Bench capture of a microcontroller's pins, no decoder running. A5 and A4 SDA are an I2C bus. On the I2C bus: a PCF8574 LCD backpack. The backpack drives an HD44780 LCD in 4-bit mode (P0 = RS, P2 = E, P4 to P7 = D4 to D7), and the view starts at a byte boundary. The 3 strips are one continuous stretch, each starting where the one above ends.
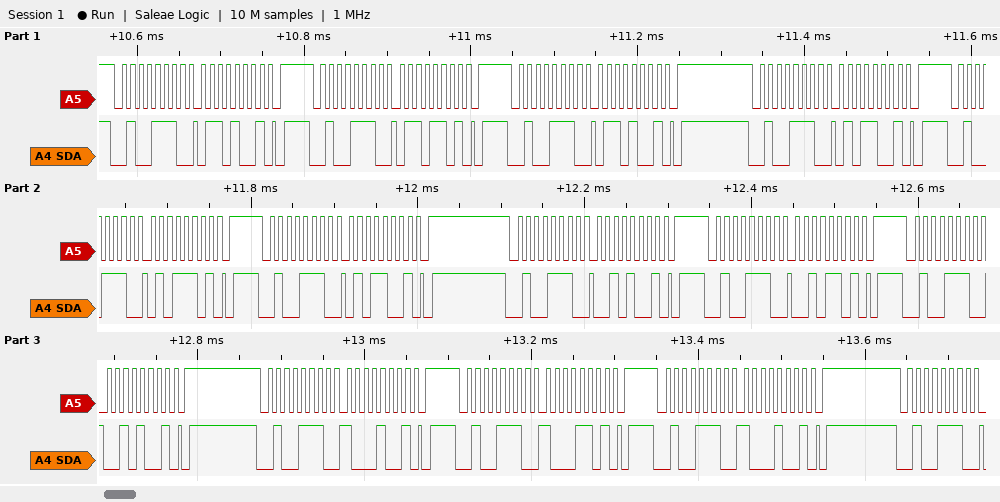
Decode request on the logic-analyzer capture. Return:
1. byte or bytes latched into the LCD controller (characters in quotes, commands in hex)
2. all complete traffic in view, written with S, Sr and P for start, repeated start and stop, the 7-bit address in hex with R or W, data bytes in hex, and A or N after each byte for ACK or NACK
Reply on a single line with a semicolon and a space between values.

'e' '('; S 27W A 69 A P S 27W A 6D A P S 27W A 69 A P S 27W A 59 A P S 27W A 5D A P S 27W A 59 A P S 27W A 29 A P S 27W A 2D A P S 27W A 29 A P S 27W A 89 A P S 27W A 8D A P S 27W A 89 A P S 27W A
